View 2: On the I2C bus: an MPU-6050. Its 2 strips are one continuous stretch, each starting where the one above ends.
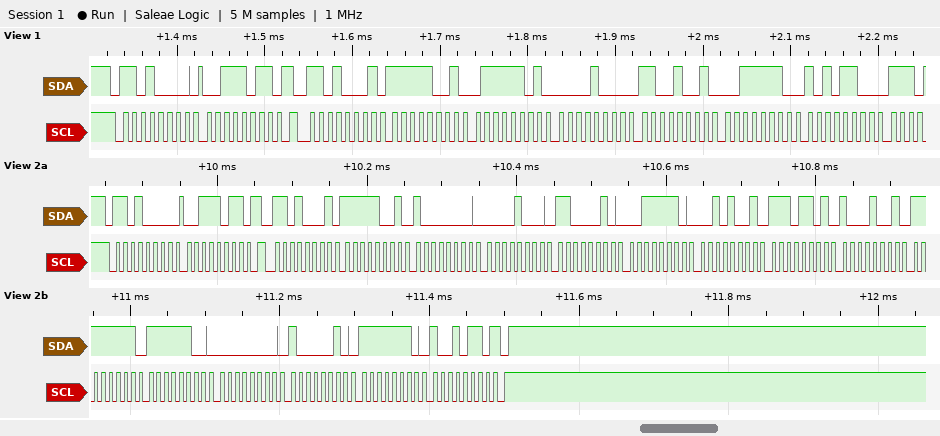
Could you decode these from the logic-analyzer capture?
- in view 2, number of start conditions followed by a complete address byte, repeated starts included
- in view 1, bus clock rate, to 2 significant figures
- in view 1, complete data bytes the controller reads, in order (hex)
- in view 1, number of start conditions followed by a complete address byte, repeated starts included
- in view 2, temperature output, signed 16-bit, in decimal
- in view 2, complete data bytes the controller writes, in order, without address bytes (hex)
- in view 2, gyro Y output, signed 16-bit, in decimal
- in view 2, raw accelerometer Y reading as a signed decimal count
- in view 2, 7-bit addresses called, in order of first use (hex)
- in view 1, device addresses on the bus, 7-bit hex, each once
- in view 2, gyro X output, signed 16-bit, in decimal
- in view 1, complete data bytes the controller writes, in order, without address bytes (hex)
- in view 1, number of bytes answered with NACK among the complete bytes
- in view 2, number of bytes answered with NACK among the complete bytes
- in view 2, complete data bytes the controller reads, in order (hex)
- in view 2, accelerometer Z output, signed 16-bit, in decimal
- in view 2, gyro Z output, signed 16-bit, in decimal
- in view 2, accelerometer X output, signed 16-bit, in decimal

2
100 kHz
F9 7D 08 C9 3E AC
2
-4727
3B
130
2242
0x68
0x68
-4
3B
0
1
F9 80 08 C2 3E 29 ED 89 FF FC 00 82 FE 96
15913
-362
-1664
